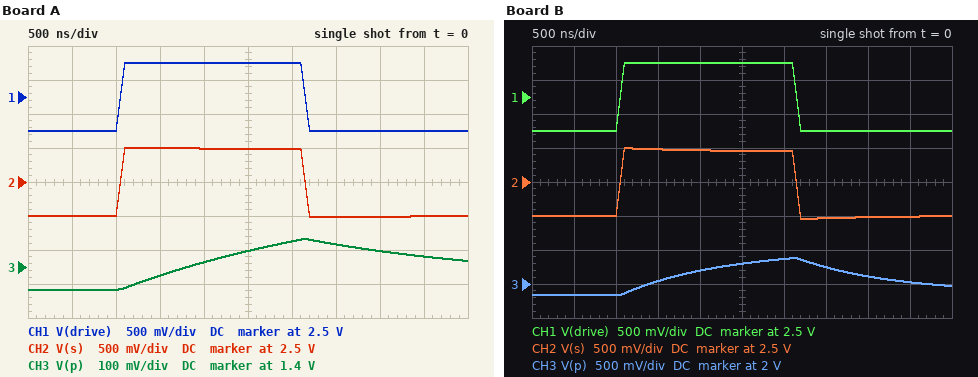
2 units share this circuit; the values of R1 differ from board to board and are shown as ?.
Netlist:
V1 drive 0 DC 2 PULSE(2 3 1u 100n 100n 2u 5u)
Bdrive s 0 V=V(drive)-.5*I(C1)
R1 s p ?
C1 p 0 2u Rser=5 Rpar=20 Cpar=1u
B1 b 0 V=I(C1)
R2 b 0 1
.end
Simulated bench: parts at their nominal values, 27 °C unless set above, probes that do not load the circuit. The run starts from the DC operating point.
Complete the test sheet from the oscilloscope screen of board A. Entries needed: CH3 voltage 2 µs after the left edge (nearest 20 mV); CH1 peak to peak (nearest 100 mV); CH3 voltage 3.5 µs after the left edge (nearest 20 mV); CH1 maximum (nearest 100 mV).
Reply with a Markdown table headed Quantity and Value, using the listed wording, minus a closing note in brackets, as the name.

| Quantity | Value |
|---|---|
| CH3 voltage 2 µs after the left edge | 1.42 V |
| CH1 peak to peak | 1.0 V |
| CH3 voltage 3.5 µs after the left edge | 1.46 V |
| CH1 maximum | 3.0 V |
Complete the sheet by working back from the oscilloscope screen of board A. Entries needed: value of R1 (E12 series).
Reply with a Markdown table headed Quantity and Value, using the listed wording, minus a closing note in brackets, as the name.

| Quantity | Value |
|---|---|
| value of R1 | 10 Ω |
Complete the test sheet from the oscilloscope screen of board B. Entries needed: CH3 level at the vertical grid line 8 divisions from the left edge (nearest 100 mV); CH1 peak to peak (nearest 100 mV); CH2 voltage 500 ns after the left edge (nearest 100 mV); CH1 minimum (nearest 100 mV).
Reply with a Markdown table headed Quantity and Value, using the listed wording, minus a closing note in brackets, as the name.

| Quantity | Value |
|---|---|
| CH3 level at the vertical grid line 8 divisions from the left edge | 2.1 V |
| CH1 peak to peak | 1.0 V |
| CH2 voltage 500 ns after the left edge | 2.0 V |
| CH1 minimum | 2.0 V |
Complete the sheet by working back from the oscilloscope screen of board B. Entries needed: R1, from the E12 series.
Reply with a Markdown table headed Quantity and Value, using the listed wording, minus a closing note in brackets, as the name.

| Quantity | Value |
|---|---|
| R1, from the E12 series | 1.8 Ω |
